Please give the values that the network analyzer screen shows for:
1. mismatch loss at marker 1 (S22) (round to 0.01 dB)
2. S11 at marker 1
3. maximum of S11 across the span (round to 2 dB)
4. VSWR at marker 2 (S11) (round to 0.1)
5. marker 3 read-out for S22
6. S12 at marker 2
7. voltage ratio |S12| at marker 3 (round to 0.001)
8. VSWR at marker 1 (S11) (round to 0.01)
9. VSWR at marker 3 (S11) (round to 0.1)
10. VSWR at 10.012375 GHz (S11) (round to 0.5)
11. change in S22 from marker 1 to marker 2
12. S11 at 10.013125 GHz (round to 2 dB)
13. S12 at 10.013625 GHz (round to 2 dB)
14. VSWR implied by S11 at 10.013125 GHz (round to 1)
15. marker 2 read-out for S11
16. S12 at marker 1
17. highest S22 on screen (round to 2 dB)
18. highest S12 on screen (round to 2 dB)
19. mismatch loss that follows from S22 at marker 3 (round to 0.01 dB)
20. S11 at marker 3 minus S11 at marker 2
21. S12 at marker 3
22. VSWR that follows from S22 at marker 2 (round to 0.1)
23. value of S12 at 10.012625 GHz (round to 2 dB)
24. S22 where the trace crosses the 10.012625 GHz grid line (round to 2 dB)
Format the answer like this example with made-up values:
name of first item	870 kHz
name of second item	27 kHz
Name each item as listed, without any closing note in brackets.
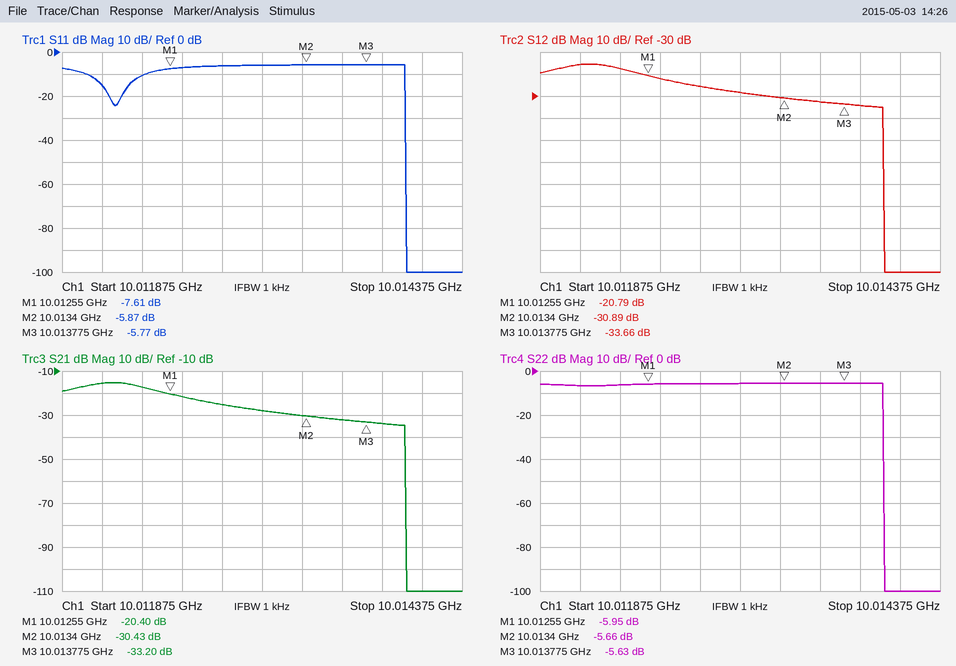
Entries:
mismatch loss at marker 1 (S22)	1.27 dB
S11 at marker 1	-7.61 dB
maximum of S11 across the span	-6 dB
VSWR at marker 2 (S11)	3.1
marker 3 read-out for S22	-5.63 dB
S12 at marker 2	-30.89 dB
voltage ratio |S12| at marker 3	0.021
VSWR at marker 1 (S11)	2.43
VSWR at marker 3 (S11)	3.1
VSWR at 10.012375 GHz (S11)	2.0
change in S22 from marker 1 to marker 2	0.29 dB
S11 at 10.013125 GHz	-6 dB
S12 at 10.013625 GHz	-32 dB
VSWR implied by S11 at 10.013125 GHz	3
marker 2 read-out for S11	-5.87 dB
S12 at marker 1	-20.79 dB
highest S22 on screen	-6 dB
highest S12 on screen	-16 dB
mismatch loss that follows from S22 at marker 3	1.39 dB
S11 at marker 3 minus S11 at marker 2	0.10 dB
S12 at marker 3	-33.66 dB
VSWR that follows from S22 at marker 2	3.2
value of S12 at 10.012625 GHz	-22 dB
S22 where the trace crosses the 10.012625 GHz grid line	-6 dB
